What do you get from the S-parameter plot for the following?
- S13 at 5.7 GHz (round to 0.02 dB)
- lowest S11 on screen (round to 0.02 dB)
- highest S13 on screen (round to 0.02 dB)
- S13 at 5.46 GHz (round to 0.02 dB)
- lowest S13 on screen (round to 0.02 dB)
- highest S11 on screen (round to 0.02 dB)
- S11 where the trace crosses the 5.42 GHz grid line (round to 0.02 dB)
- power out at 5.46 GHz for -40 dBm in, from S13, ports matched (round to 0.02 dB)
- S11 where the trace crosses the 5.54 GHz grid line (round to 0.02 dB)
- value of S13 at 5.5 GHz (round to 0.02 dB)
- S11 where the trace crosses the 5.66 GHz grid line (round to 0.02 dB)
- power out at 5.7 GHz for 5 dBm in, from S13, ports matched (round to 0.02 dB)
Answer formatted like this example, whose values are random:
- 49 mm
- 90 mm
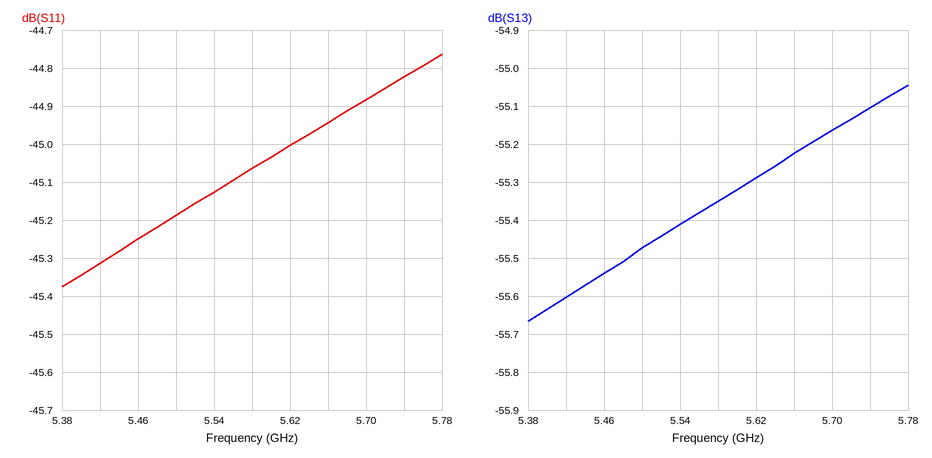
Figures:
- -55.16 dB
- -45.38 dB
- -55.04 dB
- -55.54 dB
- -55.66 dB
- -44.76 dB
- -45.32 dB
- -95.54 dBm
- -45.12 dB
- -55.48 dB
- -44.94 dB
- -50.16 dBm
